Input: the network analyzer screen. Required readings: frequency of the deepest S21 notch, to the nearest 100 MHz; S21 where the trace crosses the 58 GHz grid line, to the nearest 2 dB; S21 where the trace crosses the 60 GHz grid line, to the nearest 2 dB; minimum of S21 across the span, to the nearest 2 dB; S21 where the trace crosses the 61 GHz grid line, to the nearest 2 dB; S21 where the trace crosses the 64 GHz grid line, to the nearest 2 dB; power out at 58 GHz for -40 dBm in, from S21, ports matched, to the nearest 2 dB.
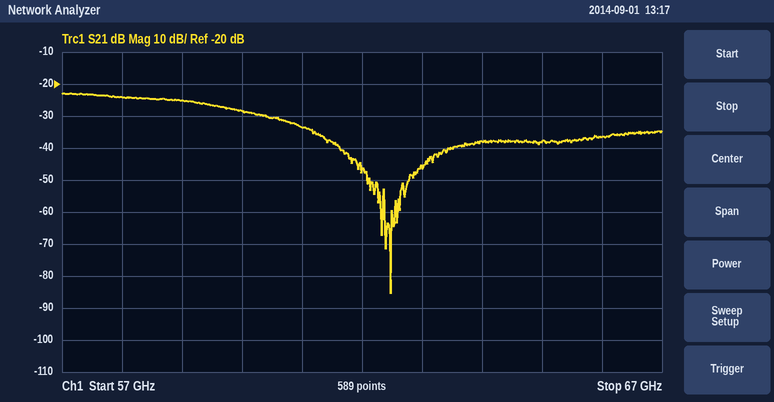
62.5 GHz
-24 dB
-28 dB
-86 dB
-34 dB
-38 dB
-64 dBm
